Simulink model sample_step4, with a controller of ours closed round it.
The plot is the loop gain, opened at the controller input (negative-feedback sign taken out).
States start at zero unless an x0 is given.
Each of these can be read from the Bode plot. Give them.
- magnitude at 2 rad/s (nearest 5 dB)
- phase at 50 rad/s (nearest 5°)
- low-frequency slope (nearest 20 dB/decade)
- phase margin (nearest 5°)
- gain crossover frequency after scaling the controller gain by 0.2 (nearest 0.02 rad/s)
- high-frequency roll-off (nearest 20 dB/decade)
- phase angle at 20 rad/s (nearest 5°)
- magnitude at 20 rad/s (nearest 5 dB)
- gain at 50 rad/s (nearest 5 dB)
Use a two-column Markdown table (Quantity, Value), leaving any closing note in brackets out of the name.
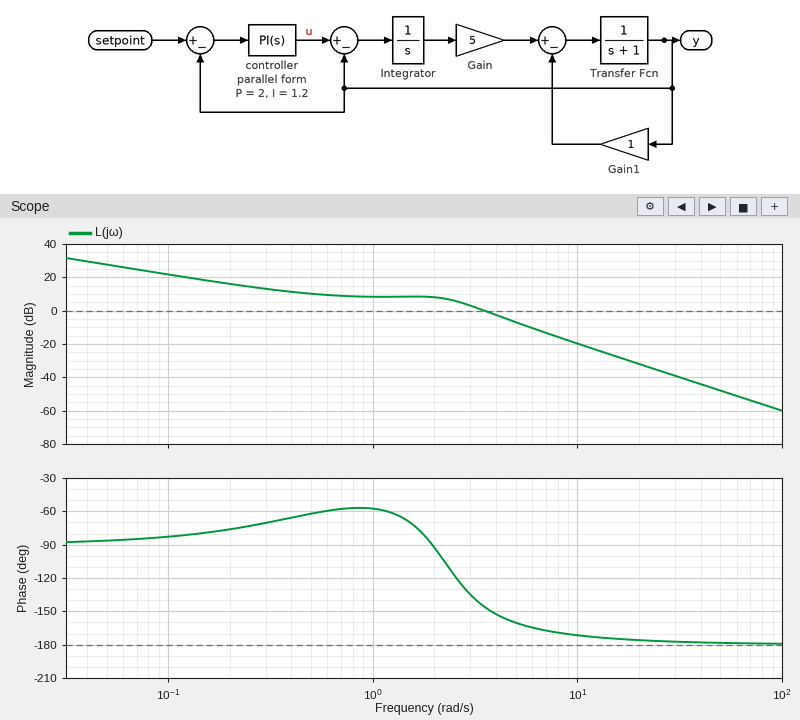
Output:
| Quantity | Value |
|---|---|
| magnitude at 2 rad/s | 10 dB |
| phase at 50 rad/s | -180° |
| low-frequency slope | -20 dB/decade |
| phase margin | 35° |
| gain crossover frequency after scaling the controller gain by 0.2 | 0.26 rad/s |
| high-frequency roll-off | -40 dB/decade |
| phase angle at 20 rad/s | -175° |
| magnitude at 20 rad/s | -30 dB |
| gain at 50 rad/s | -50 dB |
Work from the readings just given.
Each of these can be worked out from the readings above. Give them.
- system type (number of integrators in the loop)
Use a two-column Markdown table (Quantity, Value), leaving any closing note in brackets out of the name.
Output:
| Quantity | Value |
|---|---|
| system type | 1 |
